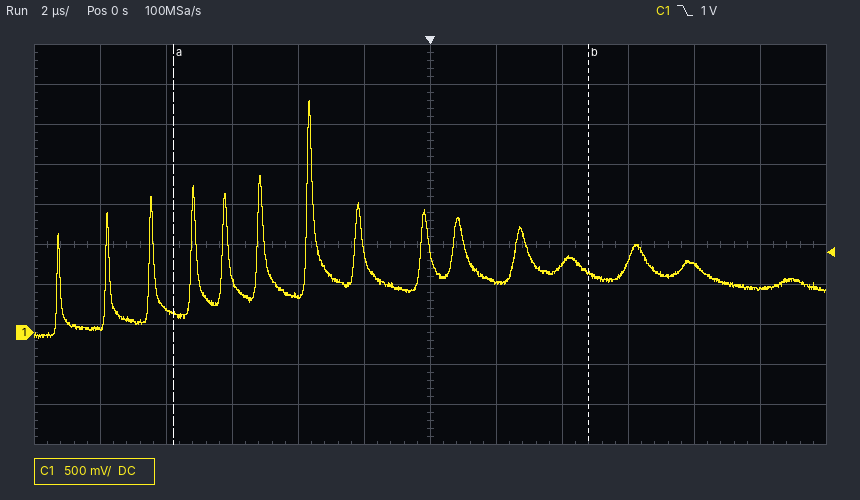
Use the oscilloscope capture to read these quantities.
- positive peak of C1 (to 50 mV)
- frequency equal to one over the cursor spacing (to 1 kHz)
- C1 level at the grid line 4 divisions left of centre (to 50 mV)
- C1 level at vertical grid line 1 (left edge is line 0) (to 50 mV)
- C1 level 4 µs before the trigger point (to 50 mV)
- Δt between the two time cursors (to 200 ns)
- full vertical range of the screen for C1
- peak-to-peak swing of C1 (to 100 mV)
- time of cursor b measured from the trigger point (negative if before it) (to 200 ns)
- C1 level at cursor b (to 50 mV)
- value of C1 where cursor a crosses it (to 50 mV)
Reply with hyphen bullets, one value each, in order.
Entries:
- 2.90 V
- 79 kHz
- 300 mV
- 50 mV
- 450 mV
- 12.6 µs
- 5 V
- 3.00 V
- +4.8 µs
- 750 mV
- 250 mV
